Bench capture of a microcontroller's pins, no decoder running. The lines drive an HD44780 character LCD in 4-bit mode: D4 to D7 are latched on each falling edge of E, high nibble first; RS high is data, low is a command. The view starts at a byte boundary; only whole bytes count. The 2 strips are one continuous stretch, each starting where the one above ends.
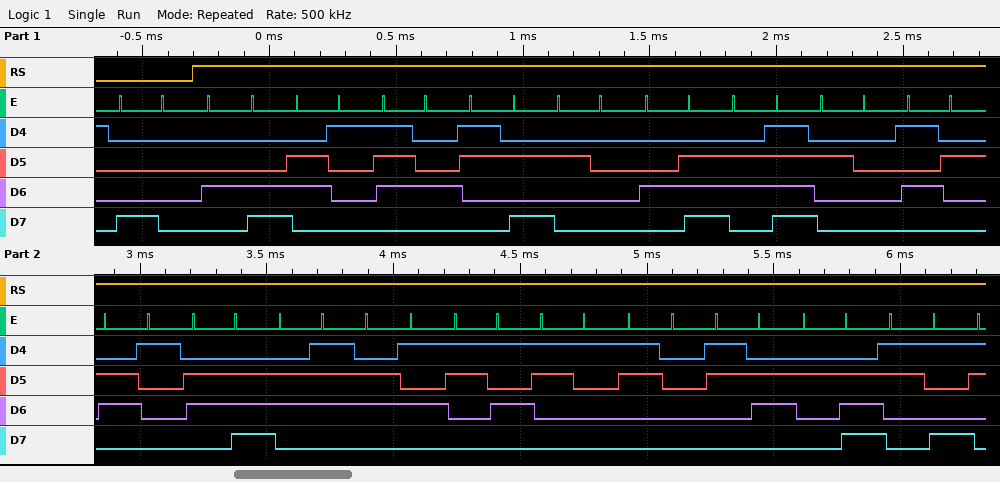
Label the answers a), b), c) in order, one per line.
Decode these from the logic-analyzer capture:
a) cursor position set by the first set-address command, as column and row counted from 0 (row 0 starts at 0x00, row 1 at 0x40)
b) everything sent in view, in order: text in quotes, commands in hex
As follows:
a) column 0, row 0
b) 0x80 "Lat: No Range5106.9"
